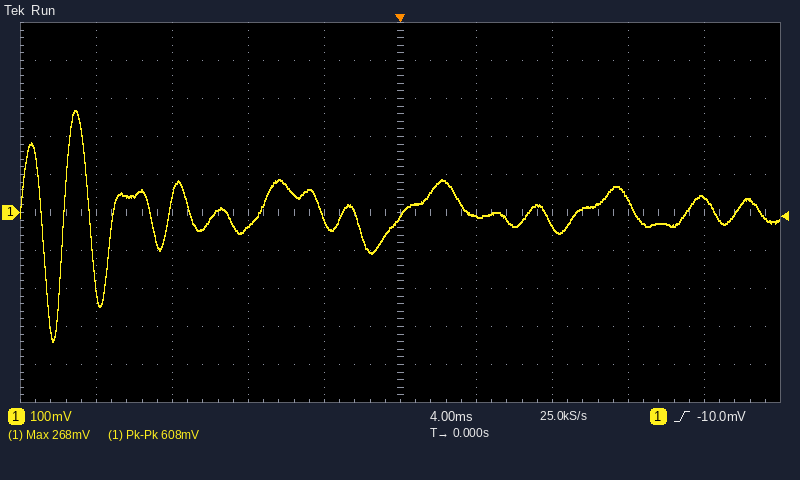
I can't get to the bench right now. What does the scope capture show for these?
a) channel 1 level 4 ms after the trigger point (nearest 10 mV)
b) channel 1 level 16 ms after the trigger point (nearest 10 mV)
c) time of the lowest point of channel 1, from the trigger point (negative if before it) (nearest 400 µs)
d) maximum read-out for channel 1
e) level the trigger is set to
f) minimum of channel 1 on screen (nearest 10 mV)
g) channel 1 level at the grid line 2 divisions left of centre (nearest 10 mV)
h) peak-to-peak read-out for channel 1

-10 mV
40 mV
-18.4 ms
268 mV
-10.0 mV
-340 mV
-40 mV
608 mV
